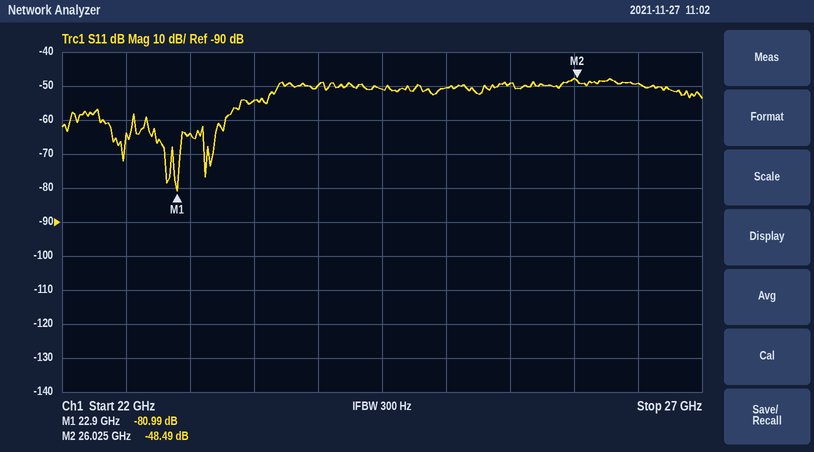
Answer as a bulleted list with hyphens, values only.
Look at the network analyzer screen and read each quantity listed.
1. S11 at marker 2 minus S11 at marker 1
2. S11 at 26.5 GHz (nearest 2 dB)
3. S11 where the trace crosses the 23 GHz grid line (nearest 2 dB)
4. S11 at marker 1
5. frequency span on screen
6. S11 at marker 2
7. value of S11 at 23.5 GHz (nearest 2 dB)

- 32.50 dB
- -50 dB
- -64 dB
- -80.99 dB
- 5 GHz
- -48.49 dB
- -54 dB
